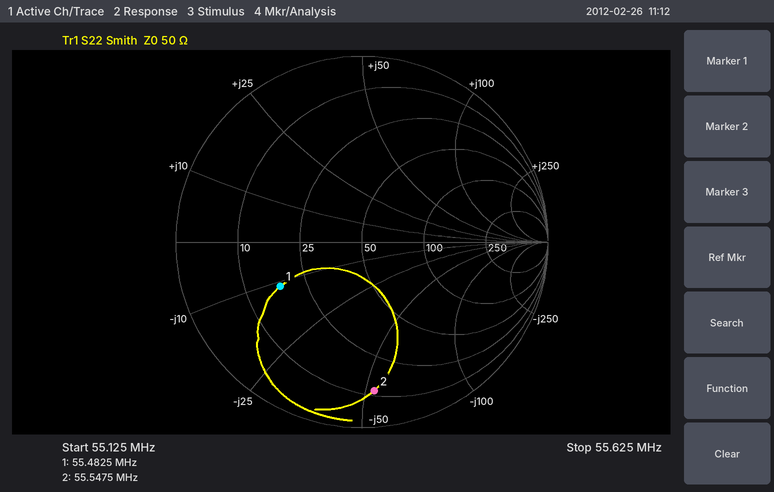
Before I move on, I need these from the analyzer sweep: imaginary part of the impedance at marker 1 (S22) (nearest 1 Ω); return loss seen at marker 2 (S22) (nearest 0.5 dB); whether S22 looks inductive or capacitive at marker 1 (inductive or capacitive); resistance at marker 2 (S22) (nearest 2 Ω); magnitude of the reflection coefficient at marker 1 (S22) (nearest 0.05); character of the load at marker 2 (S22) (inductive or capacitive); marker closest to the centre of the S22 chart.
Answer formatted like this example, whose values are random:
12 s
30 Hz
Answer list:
-11 Ω
2.0 dB
capacitive
12 Ω
0.50
capacitive
marker 1
